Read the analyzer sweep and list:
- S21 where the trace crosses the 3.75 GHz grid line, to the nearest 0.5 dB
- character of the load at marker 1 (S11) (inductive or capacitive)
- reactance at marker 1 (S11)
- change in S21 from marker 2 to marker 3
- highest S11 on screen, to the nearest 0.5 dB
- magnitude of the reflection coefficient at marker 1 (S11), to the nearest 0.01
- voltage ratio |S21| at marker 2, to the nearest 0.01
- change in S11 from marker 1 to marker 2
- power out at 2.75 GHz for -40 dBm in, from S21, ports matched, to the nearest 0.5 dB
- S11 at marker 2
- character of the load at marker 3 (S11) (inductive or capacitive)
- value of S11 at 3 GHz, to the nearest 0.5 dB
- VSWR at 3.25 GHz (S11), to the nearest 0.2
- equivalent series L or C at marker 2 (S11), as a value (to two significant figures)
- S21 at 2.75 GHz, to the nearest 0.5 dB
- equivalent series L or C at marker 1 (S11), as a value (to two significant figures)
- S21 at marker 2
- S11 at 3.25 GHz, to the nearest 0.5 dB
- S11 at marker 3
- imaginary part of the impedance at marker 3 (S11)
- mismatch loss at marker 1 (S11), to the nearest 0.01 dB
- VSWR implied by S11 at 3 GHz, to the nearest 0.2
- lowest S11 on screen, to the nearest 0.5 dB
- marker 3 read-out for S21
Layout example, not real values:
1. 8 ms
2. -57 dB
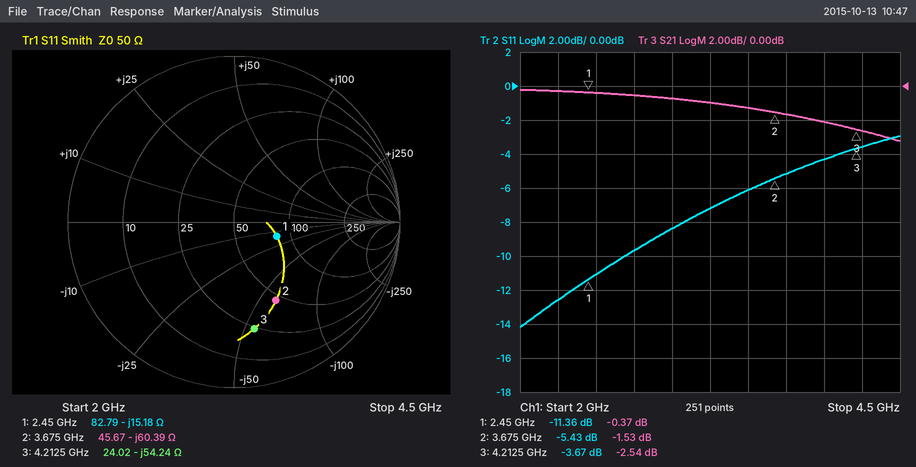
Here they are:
1. -1.5 dB
2. capacitive
3. -15.18 Ω
4. -1.01 dB
5. -3.0 dB
6. 0.27
7. 0.84
8. 5.93 dB
9. -40.5 dBm
10. -5.43 dB
11. capacitive
12. -8.5 dB
13. 2.6
14. 720 fF
15. -0.5 dB
16. 4.3 pF
17. -1.53 dB
18. -7.0 dB
19. -3.67 dB
20. -54.24 Ω
21. 0.33 dB
22. 2.2
23. -14.0 dB
24. -2.54 dB
